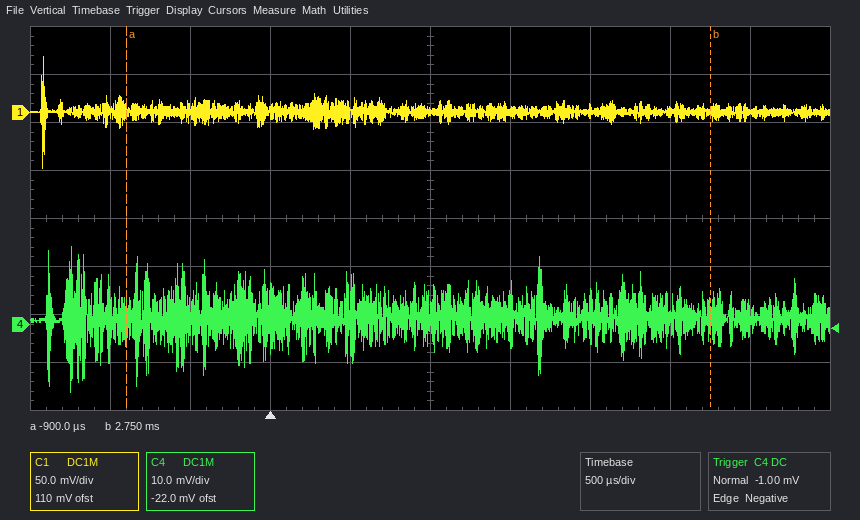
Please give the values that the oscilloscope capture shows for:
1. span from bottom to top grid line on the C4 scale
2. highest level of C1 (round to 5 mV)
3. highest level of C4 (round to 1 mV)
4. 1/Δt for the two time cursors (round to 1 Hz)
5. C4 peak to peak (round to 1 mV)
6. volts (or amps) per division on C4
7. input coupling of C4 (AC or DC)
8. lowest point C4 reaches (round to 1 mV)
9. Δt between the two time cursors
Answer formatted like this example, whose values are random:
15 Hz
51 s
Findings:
80 mV
60 mV
16 mV
274 Hz
30 mV
10 mV
DC
-14 mV
3.65 ms
